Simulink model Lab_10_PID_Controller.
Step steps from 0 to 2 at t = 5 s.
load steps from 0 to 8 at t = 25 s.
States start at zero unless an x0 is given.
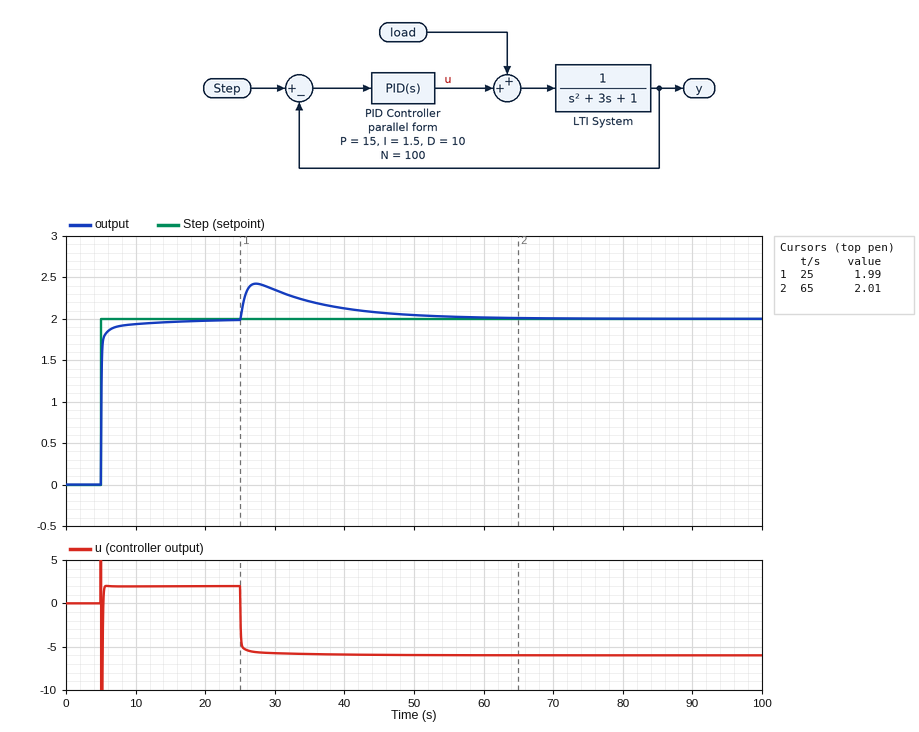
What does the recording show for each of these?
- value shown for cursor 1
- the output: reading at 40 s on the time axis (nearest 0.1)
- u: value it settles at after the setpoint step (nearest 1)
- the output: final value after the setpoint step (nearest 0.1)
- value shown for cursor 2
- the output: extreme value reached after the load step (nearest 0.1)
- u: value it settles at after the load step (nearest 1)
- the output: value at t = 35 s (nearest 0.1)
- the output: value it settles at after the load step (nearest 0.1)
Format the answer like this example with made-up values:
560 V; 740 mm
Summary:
1.99; 2.1; 2; 2.0; 2.01; 2.4; -6; 2.2; 2.0
